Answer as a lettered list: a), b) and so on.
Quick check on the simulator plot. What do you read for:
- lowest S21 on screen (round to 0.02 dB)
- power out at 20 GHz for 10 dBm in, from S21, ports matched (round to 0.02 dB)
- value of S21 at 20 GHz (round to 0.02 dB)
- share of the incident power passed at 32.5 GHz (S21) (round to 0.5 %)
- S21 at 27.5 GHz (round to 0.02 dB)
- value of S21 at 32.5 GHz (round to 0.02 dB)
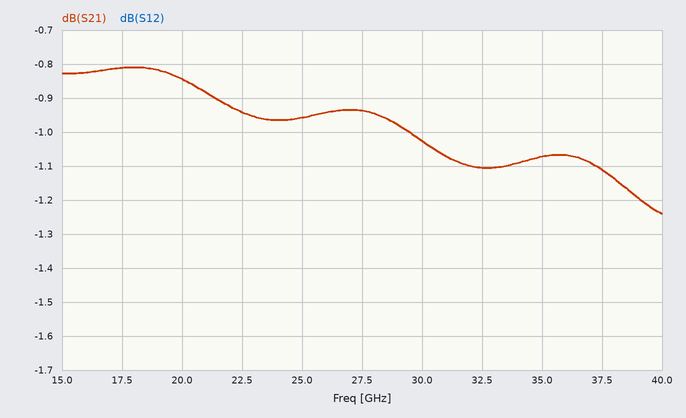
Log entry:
a) -1.24 dB
b) 9.16 dBm
c) -0.84 dB
d) 77.5 %
e) -0.94 dB
f) -1.10 dB
